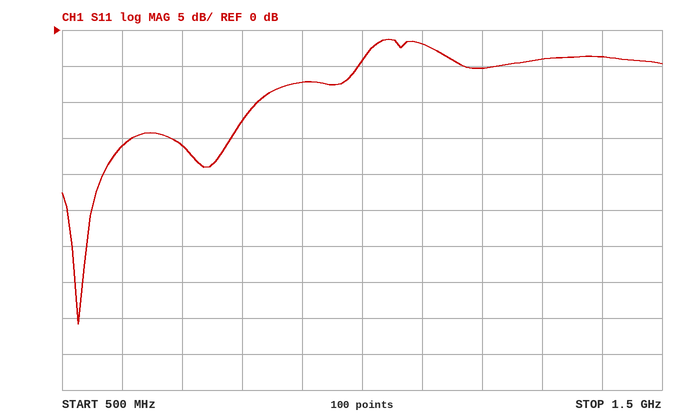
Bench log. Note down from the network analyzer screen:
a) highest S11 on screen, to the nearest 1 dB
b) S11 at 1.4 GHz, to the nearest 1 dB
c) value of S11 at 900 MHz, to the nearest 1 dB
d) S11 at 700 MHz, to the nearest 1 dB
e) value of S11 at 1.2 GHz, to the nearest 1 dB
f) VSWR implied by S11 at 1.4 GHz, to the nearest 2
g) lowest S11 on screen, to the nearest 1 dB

-1 dB
-4 dB
-7 dB
-16 dB
-5 dB
4
-41 dB
